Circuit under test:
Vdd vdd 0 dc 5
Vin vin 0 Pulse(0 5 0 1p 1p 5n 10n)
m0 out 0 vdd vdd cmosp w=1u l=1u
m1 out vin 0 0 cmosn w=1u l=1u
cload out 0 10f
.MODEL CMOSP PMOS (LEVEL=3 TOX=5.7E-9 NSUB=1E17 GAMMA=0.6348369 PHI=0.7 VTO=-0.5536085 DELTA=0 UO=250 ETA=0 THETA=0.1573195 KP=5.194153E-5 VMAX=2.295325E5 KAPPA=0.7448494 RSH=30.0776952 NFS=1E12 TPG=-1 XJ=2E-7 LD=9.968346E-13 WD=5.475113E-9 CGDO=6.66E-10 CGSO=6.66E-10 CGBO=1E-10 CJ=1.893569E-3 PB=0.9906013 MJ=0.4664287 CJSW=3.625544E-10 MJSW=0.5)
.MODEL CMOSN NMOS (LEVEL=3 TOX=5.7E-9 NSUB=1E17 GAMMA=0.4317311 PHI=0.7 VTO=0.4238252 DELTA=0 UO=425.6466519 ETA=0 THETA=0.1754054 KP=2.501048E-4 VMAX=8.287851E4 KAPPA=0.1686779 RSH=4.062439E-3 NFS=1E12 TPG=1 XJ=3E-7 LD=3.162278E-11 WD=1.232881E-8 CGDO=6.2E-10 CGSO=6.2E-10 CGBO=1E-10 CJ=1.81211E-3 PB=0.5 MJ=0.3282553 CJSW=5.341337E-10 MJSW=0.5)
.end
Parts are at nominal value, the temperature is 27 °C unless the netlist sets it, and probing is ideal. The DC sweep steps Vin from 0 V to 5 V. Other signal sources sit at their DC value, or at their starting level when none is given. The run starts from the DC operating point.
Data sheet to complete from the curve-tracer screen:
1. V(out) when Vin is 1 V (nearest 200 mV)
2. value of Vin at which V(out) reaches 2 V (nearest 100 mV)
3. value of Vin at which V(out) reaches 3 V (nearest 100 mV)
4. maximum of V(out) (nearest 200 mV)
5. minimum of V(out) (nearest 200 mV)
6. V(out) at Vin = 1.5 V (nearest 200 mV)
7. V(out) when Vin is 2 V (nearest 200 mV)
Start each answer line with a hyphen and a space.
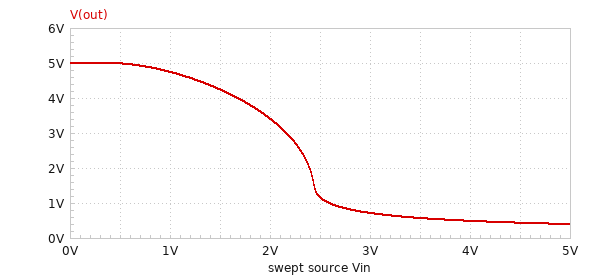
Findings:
- 4.8 V
- 2.4 V
- 2.2 V
- 5.0 V
- 400 mV
- 4.2 V
- 3.4 V
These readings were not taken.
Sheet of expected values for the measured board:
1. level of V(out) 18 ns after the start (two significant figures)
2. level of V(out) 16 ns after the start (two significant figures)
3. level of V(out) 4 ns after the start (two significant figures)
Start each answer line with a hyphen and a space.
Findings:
- 5.0 V
- 5.0 V
- 400 mV
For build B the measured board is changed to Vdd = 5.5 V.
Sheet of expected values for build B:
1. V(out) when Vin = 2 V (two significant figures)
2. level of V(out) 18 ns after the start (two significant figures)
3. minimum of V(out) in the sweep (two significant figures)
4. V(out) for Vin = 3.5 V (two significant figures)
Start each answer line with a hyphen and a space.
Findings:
- 4.1 V
- 5.5 V
- 480 mV
- 720 mV
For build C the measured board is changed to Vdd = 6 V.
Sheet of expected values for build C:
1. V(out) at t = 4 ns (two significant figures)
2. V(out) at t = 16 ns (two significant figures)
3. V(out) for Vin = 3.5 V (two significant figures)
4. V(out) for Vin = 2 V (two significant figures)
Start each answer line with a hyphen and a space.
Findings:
- 570 mV
- 6.0 V
- 890 mV
- 4.7 V
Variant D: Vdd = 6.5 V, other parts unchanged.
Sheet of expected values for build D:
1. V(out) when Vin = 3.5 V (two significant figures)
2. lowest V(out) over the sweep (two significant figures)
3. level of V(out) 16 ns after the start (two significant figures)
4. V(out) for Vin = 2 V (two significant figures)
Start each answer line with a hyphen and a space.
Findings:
- 1.1 V
- 670 mV
- 6.5 V
- 5.3 V
